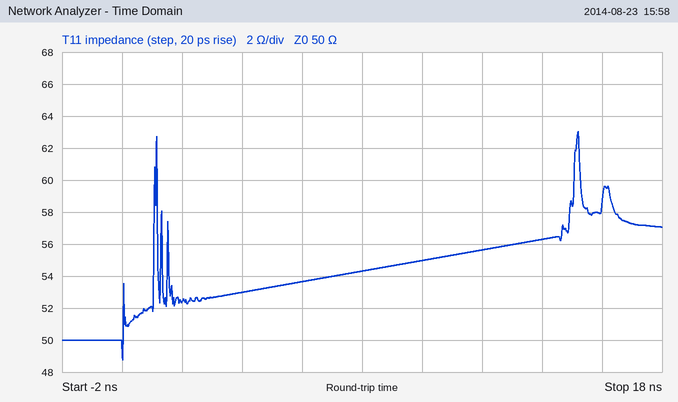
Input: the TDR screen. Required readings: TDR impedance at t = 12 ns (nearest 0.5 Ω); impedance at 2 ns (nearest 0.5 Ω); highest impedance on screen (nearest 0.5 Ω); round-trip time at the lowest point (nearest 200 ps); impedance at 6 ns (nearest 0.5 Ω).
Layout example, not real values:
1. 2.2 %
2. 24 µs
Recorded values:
1. 55.5 Ω
2. 52.5 Ω
3. 63.0 Ω
4. 0.0 ns
5. 53.5 Ω
